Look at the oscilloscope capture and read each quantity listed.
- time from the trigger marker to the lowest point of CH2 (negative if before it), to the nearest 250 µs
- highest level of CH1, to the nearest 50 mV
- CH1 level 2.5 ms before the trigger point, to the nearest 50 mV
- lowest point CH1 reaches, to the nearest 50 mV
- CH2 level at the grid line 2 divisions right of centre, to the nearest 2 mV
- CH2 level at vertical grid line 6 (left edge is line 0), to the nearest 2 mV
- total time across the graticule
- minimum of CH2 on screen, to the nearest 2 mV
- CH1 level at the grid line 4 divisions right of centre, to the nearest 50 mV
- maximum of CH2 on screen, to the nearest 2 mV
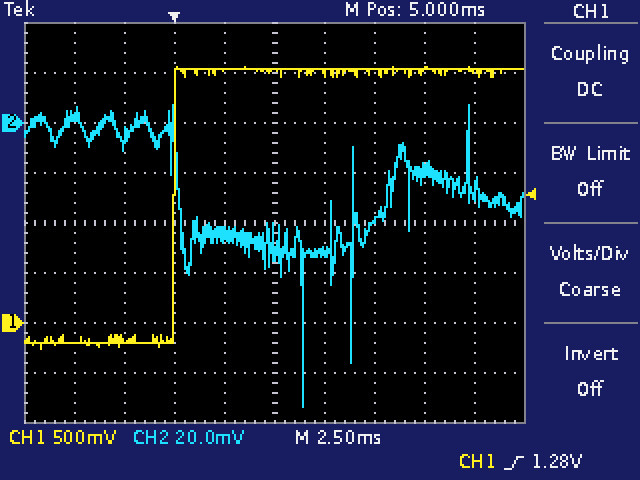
+6.50 ms
2.55 V
-150 mV
-250 mV
-40 mV
-52 mV
25 ms
-114 mV
2.50 V
8 mV
